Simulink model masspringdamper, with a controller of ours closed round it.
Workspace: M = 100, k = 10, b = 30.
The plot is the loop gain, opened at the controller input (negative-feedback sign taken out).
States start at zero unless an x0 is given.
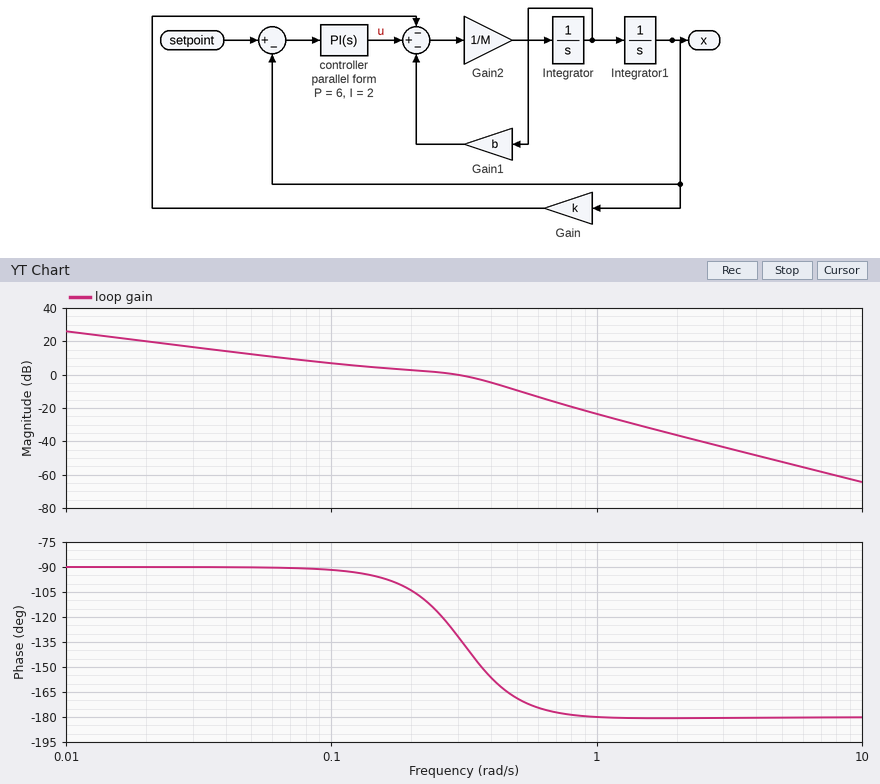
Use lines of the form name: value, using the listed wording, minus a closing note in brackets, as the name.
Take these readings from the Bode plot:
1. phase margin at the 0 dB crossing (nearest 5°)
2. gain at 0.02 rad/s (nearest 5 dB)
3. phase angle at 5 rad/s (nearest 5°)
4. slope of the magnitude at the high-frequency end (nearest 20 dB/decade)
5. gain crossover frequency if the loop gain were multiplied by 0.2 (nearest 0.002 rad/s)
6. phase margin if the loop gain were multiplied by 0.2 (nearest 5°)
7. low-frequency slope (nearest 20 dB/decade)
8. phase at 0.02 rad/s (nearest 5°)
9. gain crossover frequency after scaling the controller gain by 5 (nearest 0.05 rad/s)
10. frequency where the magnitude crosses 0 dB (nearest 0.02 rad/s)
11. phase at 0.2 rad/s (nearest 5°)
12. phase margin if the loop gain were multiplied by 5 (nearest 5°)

phase margin at the 0 dB crossing: 50°
gain at 0.02 rad/s: 20 dB
phase angle at 5 rad/s: -180°
slope of the magnitude at the high-frequency end: -40 dB/decade
gain crossover frequency if the loop gain were multiplied by 0.2: 0.040 rad/s
phase margin if the loop gain were multiplied by 0.2: 90°
low-frequency slope: -20 dB/decade
phase at 0.02 rad/s: -90°
gain crossover frequency after scaling the controller gain by 5: 0.60 rad/s
frequency where the magnitude crosses 0 dB: 0.30 rad/s
phase at 0.2 rad/s: -105°
phase margin if the loop gain were multiplied by 5: 5°
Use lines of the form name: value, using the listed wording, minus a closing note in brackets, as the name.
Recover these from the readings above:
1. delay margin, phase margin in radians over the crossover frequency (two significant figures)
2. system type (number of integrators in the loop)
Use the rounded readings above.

delay margin, phase margin in radians over the crossover frequency: 2.9 s
system type: 1
